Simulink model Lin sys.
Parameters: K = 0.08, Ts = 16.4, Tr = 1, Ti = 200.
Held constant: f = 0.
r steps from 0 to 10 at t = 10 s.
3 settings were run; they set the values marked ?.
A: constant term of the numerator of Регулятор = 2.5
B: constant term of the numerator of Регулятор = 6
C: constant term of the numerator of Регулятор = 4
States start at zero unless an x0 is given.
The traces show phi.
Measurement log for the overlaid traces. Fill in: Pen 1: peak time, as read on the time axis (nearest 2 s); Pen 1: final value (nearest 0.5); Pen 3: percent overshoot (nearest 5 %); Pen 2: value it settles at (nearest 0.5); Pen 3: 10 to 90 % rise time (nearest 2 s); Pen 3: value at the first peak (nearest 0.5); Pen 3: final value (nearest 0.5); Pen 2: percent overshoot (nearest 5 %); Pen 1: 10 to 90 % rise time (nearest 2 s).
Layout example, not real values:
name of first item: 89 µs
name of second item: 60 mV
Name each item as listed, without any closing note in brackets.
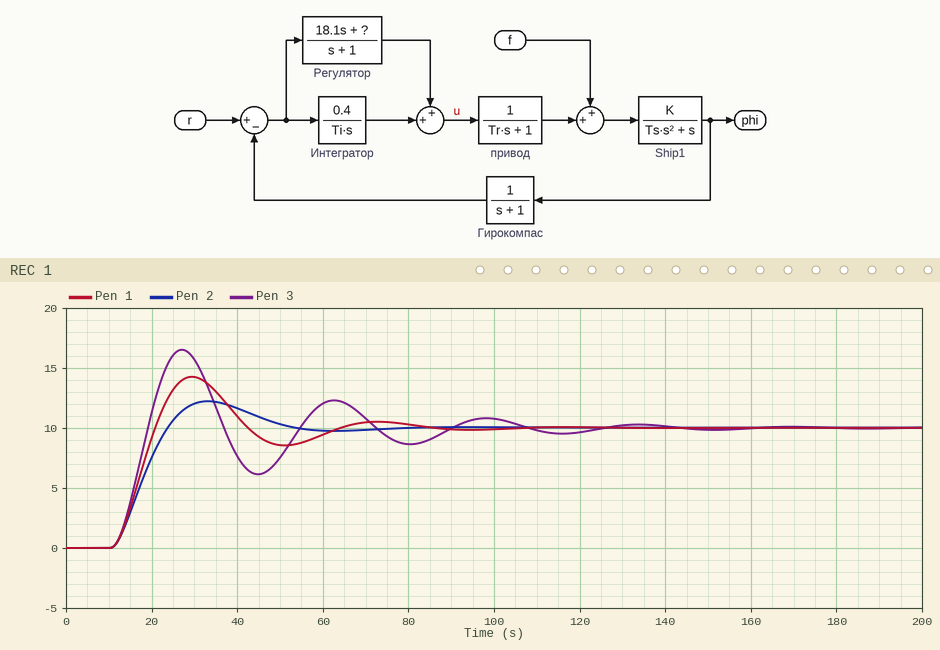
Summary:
Pen 1: peak time, as read on the time axis: 30 s
Pen 1: final value: 10.0
Pen 3: percent overshoot: 65 %
Pen 2: value it settles at: 10.0
Pen 3: 10 to 90 % rise time: 6 s
Pen 3: value at the first peak: 16.5
Pen 3: final value: 10.0
Pen 2: percent overshoot: 20 %
Pen 1: 10 to 90 % rise time: 8 s
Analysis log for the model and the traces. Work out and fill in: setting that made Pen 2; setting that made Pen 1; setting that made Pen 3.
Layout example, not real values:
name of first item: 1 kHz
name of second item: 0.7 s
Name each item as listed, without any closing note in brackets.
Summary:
setting that made Pen 2: A
setting that made Pen 1: C
setting that made Pen 3: B
